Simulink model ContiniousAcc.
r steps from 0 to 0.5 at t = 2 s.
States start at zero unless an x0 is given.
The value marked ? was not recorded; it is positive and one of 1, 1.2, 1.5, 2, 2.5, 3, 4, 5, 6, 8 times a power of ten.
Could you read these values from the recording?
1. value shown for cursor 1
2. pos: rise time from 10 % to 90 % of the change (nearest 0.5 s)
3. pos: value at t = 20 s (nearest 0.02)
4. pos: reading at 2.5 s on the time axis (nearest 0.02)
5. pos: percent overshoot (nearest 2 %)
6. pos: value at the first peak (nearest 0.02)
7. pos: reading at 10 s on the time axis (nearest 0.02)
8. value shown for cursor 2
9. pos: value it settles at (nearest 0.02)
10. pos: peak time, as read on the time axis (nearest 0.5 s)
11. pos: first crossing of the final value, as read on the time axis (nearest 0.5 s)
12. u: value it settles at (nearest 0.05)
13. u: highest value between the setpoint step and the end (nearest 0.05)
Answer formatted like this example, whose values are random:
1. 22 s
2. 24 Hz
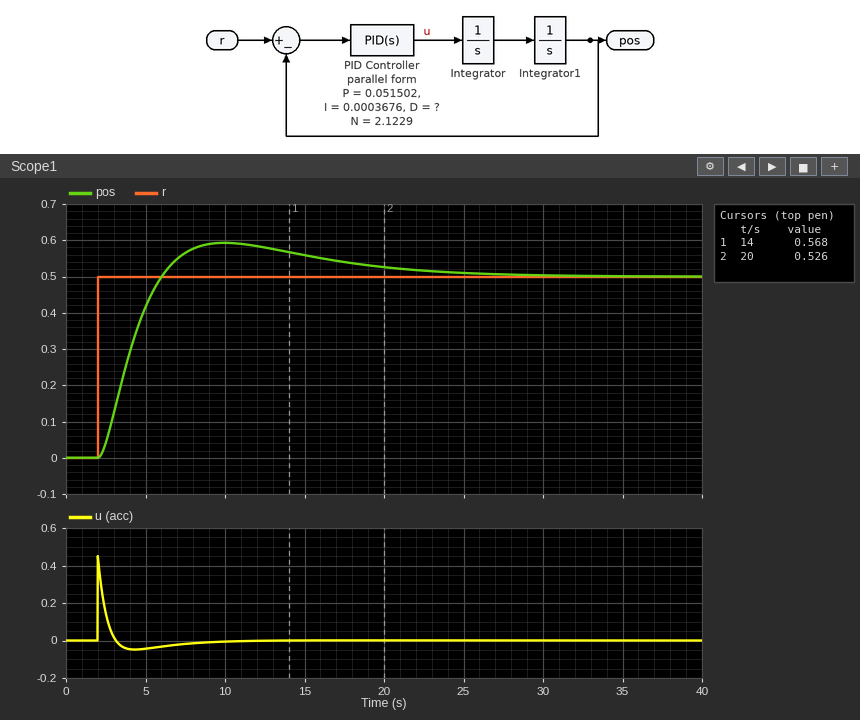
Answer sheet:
1. 0.568
2. 3.0 s
3. 0.52
4. 0.04
5. 18 %
6. 0.60
7. 0.60
8. 0.526
9. 0.50
10. 10.0 s
11. 6.0 s
12. 0.00
13. 0.45
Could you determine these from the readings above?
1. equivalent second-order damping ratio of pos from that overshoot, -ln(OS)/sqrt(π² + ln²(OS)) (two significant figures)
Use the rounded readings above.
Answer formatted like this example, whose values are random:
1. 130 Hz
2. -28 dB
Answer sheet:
1. 0.48
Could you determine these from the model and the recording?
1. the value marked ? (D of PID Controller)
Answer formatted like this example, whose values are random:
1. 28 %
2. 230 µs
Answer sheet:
1. 0.4
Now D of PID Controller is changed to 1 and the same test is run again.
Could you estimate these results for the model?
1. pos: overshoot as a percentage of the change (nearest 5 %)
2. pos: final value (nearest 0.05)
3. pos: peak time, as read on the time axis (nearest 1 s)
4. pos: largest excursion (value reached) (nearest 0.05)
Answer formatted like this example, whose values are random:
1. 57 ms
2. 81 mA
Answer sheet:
1. 10 %
2. 0.50
3. 5 s
4. 0.55
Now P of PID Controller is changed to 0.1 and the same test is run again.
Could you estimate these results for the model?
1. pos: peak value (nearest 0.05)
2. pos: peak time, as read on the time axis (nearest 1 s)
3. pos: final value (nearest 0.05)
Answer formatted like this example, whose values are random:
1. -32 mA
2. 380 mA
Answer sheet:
1. 0.65
2. 8 s
3. 0.50
